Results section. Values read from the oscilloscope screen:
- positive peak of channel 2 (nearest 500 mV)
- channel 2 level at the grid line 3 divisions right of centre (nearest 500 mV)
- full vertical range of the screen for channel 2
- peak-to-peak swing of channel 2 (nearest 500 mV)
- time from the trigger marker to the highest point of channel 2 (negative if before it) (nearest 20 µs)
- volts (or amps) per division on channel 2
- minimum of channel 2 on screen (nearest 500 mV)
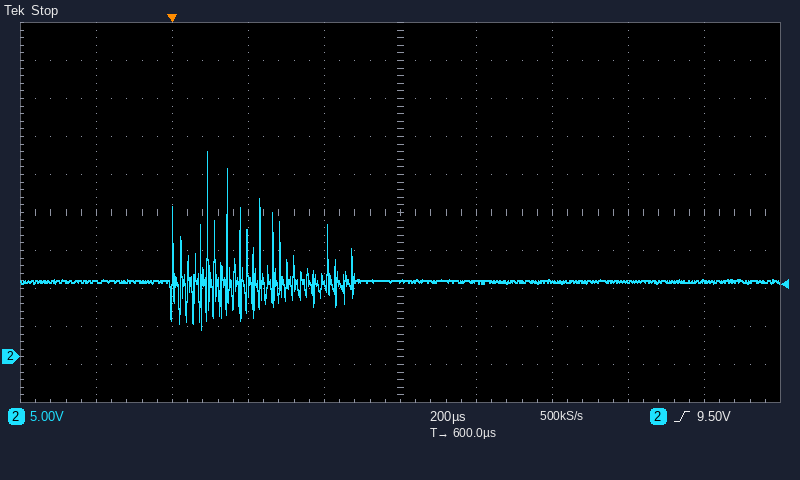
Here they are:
27.0 V
10.0 V
50 V
23.5 V
+100 µs
5 V
3.5 V
